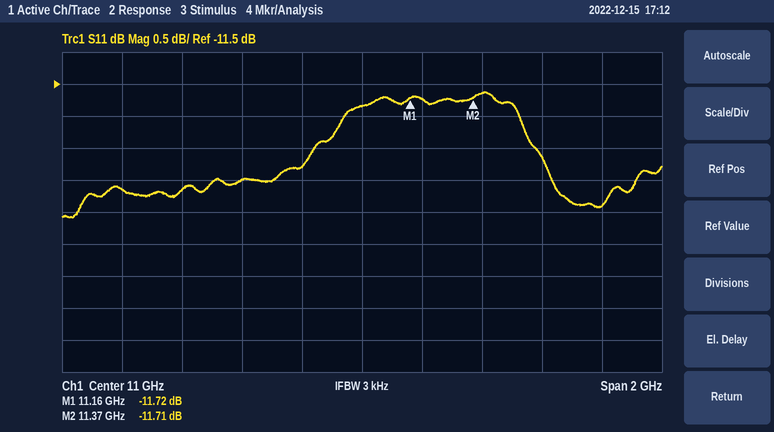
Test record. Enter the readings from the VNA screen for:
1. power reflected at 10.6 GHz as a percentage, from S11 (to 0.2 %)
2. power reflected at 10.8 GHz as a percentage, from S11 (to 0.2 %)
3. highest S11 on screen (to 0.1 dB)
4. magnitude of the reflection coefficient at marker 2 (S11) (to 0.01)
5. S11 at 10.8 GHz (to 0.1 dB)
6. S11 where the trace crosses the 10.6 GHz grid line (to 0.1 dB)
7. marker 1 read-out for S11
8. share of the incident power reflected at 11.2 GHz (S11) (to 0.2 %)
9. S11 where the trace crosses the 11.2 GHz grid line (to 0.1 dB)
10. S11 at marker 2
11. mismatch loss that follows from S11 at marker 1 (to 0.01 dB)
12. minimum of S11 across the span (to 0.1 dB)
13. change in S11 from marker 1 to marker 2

5.0 %
5.2 %
-11.6 dB
0.26
-12.8 dB
-13.0 dB
-11.72 dB
6.8 %
-11.7 dB
-11.71 dB
0.30 dB
-13.6 dB
0.01 dB
